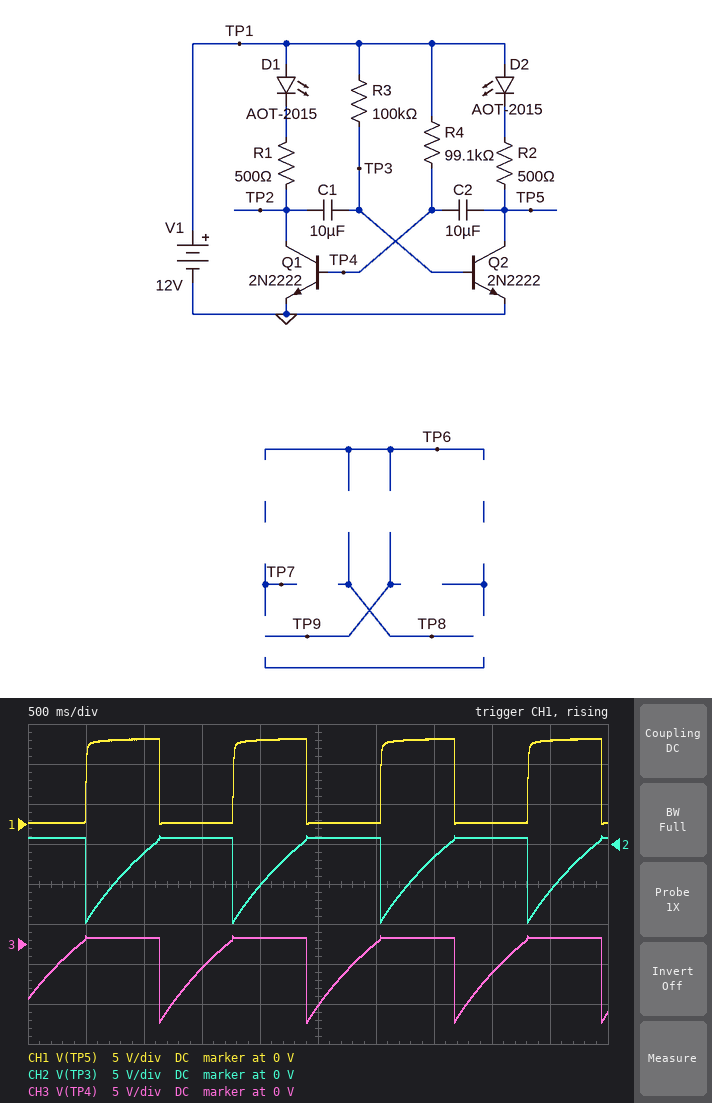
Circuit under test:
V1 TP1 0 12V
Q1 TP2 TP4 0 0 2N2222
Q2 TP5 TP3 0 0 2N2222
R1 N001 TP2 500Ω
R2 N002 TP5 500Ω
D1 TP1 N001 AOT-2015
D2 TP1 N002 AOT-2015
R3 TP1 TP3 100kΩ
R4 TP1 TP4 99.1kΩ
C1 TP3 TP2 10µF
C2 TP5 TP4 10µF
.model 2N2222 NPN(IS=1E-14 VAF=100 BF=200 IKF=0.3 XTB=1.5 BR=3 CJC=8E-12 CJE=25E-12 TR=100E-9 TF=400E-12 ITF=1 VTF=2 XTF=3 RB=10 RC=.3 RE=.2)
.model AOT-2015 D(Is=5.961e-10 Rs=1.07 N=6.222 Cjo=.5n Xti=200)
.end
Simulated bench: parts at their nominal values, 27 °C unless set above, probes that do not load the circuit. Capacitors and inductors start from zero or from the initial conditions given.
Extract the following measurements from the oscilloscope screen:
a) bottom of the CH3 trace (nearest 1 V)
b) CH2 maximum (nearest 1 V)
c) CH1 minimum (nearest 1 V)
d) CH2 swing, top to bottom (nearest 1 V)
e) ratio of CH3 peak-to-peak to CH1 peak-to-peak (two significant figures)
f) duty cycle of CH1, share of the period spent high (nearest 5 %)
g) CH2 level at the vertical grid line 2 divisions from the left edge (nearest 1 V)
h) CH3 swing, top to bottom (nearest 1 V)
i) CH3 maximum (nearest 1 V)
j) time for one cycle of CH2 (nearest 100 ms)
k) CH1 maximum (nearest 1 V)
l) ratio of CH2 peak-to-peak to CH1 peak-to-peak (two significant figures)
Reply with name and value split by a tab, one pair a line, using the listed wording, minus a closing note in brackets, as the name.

bottom of the CH3 trace	-10 V
CH2 maximum	1 V
CH1 minimum	0 V
CH2 swing, top to bottom	11 V
ratio of CH3 peak-to-peak to CH1 peak-to-peak	1.0
duty cycle of CH1, share of the period spent high	50 %
CH2 level at the vertical grid line 2 divisions from the left edge	-1 V
CH3 swing, top to bottom	11 V
CH3 maximum	1 V
time for one cycle of CH2	1.3 s
CH1 maximum	11 V
ratio of CH2 peak-to-peak to CH1 peak-to-peak	1.0
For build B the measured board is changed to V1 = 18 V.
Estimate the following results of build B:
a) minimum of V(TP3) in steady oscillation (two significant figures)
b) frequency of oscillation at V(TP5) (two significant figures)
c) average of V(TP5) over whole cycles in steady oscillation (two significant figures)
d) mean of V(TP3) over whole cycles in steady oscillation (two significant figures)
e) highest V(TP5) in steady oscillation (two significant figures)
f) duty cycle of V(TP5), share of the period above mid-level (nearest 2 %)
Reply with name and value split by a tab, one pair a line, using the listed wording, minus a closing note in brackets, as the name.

minimum of V(TP3) in steady oscillation	-16 V
frequency of oscillation at V(TP5)	770 mHz
average of V(TP5) over whole cycles in steady oscillation	8.3 V
mean of V(TP3) over whole cycles in steady oscillation	-3.0 V
highest V(TP5) in steady oscillation	17 V
duty cycle of V(TP5), share of the period above mid-level	50 %
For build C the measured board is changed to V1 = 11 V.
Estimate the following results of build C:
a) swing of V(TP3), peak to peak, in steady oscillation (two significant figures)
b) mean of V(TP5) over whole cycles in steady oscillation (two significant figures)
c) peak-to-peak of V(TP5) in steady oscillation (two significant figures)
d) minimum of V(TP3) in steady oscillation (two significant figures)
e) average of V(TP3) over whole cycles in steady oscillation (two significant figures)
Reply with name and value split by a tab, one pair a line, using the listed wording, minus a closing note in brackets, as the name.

swing of V(TP3), peak to peak, in steady oscillation	9.8 V
mean of V(TP5) over whole cycles in steady oscillation	4.8 V
peak-to-peak of V(TP5) in steady oscillation	9.6 V
minimum of V(TP3) in steady oscillation	-8.9 V
average of V(TP3) over whole cycles in steady oscillation	-1.5 V
